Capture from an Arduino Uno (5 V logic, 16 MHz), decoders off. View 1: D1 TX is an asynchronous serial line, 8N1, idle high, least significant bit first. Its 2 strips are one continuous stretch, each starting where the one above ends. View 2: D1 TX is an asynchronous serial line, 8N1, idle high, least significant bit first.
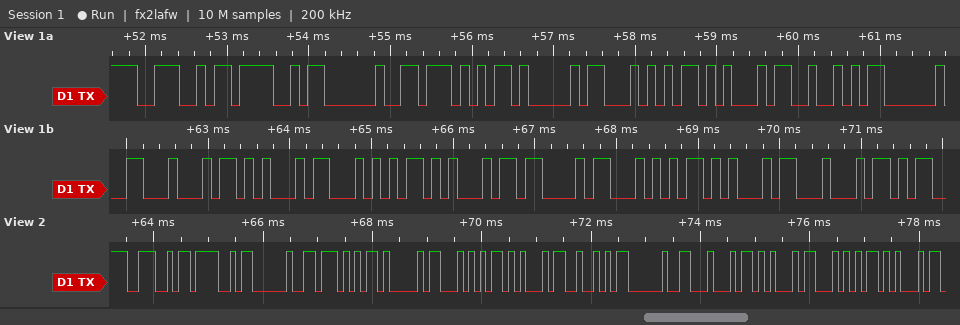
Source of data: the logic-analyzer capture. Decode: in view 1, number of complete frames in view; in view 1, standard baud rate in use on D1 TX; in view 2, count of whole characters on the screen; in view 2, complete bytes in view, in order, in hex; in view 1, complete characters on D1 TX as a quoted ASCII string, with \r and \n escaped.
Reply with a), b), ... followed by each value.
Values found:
a) 17
b) 9600 baud
c) 13
d) 0x4E 0x4F 0x20 0x57 0x41 0x54 0x45 0x52 0x20 0x44 0x45 0x54 0x45
e) "NO WATER DETECTED"
